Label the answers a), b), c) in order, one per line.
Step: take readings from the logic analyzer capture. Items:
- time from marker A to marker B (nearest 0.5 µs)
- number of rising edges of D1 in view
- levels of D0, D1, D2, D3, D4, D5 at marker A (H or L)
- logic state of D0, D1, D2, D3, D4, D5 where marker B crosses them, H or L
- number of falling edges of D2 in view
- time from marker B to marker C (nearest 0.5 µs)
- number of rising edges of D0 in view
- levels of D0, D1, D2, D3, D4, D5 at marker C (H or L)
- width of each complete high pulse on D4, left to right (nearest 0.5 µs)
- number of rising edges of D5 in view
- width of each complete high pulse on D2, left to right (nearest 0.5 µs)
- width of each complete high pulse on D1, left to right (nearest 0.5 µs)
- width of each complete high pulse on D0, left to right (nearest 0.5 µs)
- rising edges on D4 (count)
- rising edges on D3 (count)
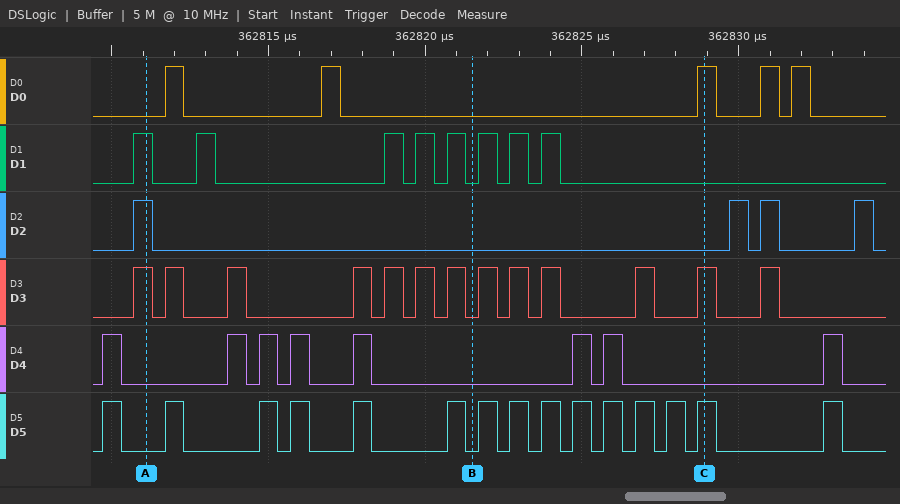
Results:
a) 10.5 µs
b) 8
c) D0=L, D1=H, D2=H, D3=H, D4=L, D5=L
d) D0=L, D1=L, D2=L, D3=L, D4=L, D5=L
e) 4
f) 7.5 µs
g) 5
h) D0=H, D1=L, D2=L, D3=H, D4=L, D5=H
i) 0.5 µs, 0.5 µs, 0.5 µs, 0.5 µs, 0.5 µs, 0.5 µs, 0.5 µs, 0.5 µs
j) 15
k) 0.5 µs, 0.5 µs, 0.5 µs, 0.5 µs
l) 0.5 µs, 0.5 µs, 0.5 µs, 0.5 µs, 0.5 µs, 0.5 µs, 0.5 µs, 0.5 µs
m) 0.5 µs, 0.5 µs, 0.5 µs, 0.5 µs, 0.5 µs
n) 8
o) 13
